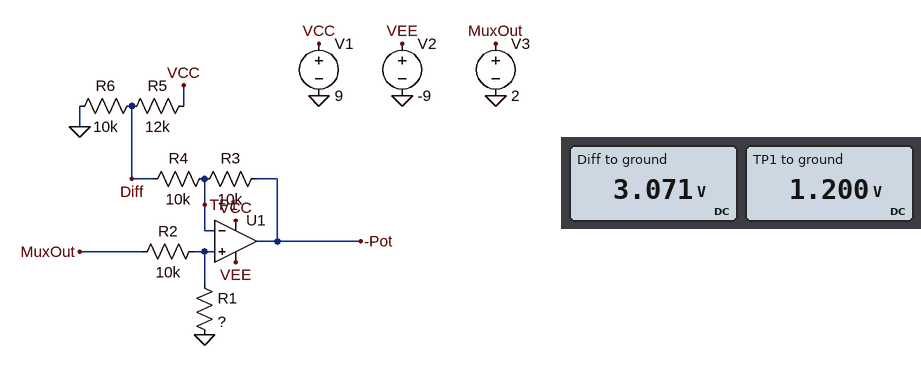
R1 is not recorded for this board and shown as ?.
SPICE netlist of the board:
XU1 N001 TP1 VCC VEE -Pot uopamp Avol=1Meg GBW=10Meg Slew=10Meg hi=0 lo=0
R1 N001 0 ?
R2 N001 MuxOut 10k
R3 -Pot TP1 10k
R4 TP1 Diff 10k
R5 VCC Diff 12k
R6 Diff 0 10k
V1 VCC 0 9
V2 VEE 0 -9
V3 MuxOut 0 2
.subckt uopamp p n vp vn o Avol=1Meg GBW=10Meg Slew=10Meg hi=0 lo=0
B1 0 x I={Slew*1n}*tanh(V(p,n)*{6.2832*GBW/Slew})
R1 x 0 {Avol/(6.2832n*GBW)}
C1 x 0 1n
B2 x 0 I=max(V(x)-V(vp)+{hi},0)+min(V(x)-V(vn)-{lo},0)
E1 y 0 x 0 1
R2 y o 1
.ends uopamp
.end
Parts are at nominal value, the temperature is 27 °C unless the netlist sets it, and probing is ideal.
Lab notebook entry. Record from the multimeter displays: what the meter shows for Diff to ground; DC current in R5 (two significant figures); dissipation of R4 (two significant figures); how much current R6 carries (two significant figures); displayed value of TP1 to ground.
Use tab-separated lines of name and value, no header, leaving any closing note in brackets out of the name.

what the meter shows for Diff to ground	3.071 V
DC current in R5	490 µA
dissipation of R4	350 µW
how much current R6 carries	310 µA
displayed value of TP1 to ground	1.200 V
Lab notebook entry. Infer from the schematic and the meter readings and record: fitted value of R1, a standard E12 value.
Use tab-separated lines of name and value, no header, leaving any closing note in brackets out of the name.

fitted value of R1, a standard E12 value	15 kΩ
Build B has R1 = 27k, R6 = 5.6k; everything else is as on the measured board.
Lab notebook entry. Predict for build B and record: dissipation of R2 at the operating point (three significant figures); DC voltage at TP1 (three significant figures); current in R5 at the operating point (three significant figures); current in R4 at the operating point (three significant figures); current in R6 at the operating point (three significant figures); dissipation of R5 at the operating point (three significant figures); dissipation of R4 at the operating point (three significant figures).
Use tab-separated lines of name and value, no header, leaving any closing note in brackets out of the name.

dissipation of R2 at the operating point	29.2 µW
DC voltage at TP1	1.46 V
current in R5 at the operating point	544 µA
current in R4 at the operating point	102 µA
current in R6 at the operating point	442 µA
dissipation of R5 at the operating point	3.55 mW
dissipation of R4 at the operating point	103 µW
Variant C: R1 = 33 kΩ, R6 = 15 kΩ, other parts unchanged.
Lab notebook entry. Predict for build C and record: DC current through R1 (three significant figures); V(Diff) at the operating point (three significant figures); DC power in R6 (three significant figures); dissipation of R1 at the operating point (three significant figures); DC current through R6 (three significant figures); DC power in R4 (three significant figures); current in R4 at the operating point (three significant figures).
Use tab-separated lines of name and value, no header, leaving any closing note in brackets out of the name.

DC current through R1	46.5 µA
V(Diff) at the operating point	3.61 V
DC power in R6	871 µW
dissipation of R1 at the operating point	71.4 µW
DC current through R6	241 µA
DC power in R4	432 µW
current in R4 at the operating point	208 µA
